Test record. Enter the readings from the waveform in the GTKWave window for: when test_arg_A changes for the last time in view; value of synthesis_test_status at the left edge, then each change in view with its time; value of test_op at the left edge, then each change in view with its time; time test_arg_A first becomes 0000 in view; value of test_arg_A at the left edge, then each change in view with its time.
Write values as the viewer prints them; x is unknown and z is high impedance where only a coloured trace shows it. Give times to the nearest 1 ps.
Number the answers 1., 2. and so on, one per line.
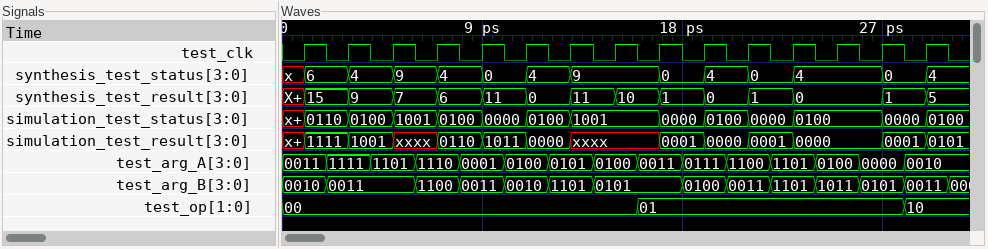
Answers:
1. 28 ps
2. x, 6 at 1 ps, 4 at 3 ps, 9 at 5 ps, 4 at 7 ps, 0 at 9 ps, 4 at 11 ps, 9 at 13 ps, 0 at 17 ps, 4 at 19 ps, 0 at 21 ps, 4 at 23 ps, 0 at 27 ps, 4 at 29 ps
3. 00, 01 at 16 ps, 10 at 28 ps
4. 26 ps
5. 0011, 1111 at 2 ps, 1101 at 4 ps, 1110 at 6 ps, 0001 at 8 ps, 0100 at 10 ps, 0101 at 12 ps, 0100 at 14 ps, 0011 at 16 ps, 0111 at 18 ps, 1100 at 20 ps, 1101 at 22 ps, 0100 at 24 ps, 0000 at 26 ps, 0010 at 28 ps
